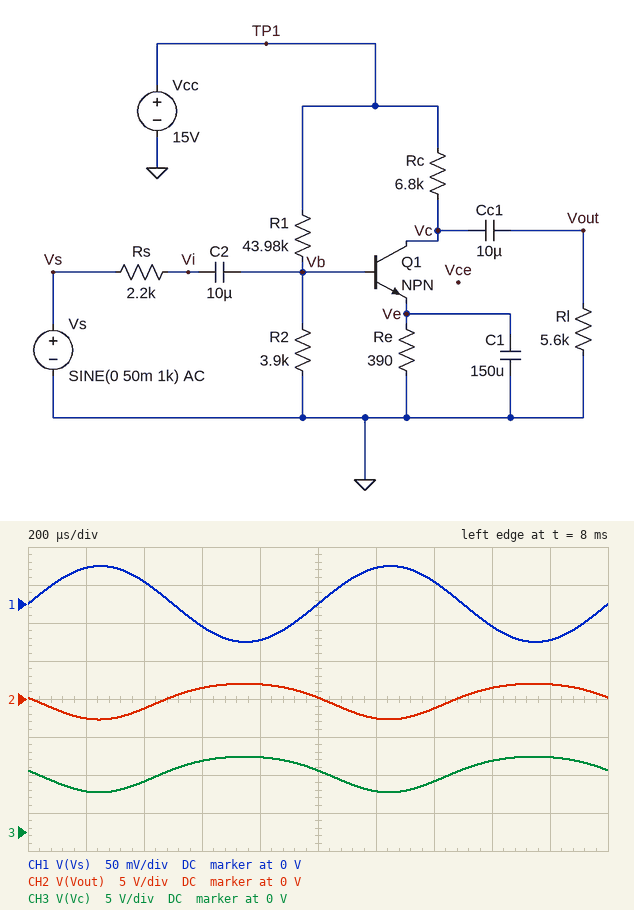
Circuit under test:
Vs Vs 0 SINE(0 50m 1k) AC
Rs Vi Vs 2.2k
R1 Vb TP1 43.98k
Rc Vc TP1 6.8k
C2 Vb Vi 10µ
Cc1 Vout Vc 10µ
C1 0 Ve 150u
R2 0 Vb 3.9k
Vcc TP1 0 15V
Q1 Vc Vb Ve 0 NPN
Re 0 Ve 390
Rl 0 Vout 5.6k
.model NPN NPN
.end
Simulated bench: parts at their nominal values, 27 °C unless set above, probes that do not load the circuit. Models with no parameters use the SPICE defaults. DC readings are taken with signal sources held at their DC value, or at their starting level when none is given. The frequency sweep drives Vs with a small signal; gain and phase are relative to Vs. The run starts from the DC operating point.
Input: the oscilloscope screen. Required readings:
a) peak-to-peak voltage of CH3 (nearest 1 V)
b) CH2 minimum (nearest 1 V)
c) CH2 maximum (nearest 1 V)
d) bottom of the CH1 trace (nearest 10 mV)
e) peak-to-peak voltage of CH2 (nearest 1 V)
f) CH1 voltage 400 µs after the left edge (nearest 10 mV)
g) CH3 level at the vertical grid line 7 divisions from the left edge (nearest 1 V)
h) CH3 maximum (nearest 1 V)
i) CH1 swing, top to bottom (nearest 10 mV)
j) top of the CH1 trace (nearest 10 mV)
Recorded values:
5 V
-3 V
2 V
-50 mV
5 V
30 mV
7 V
10 V
100 mV
50 mV
